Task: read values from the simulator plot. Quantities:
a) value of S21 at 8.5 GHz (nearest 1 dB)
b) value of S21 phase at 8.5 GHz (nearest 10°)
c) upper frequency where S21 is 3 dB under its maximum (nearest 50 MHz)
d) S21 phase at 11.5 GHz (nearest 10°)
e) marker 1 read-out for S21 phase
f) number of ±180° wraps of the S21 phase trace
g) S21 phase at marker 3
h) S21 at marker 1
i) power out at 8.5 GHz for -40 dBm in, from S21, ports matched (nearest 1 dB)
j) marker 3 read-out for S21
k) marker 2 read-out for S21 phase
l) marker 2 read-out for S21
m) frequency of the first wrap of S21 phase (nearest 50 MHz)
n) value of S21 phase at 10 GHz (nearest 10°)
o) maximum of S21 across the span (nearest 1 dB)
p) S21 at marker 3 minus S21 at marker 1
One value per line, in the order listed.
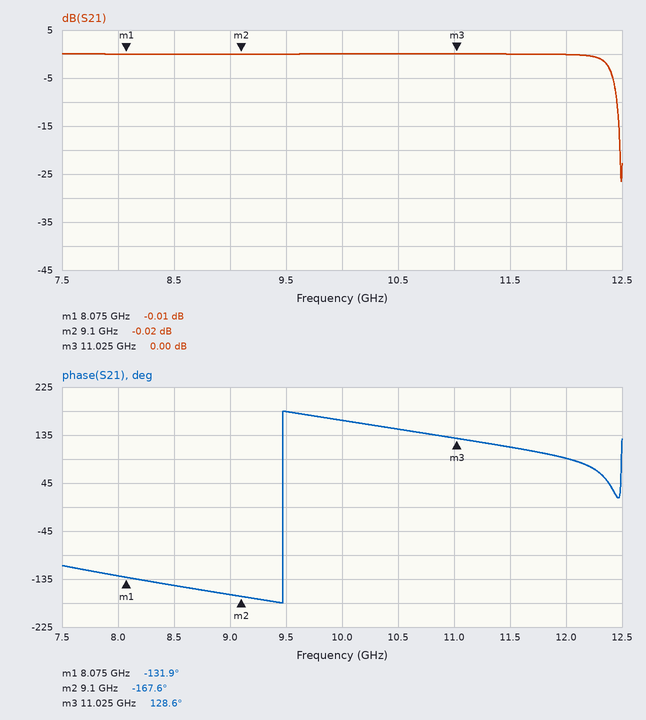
0 dB
-150°
12.40 GHz
110°
-131.9°
1
128.6°
-0.01 dB
-40 dBm
0.00 dB
-167.6°
-0.02 dB
9.45 GHz
160°
0 dB
0.01 dB
